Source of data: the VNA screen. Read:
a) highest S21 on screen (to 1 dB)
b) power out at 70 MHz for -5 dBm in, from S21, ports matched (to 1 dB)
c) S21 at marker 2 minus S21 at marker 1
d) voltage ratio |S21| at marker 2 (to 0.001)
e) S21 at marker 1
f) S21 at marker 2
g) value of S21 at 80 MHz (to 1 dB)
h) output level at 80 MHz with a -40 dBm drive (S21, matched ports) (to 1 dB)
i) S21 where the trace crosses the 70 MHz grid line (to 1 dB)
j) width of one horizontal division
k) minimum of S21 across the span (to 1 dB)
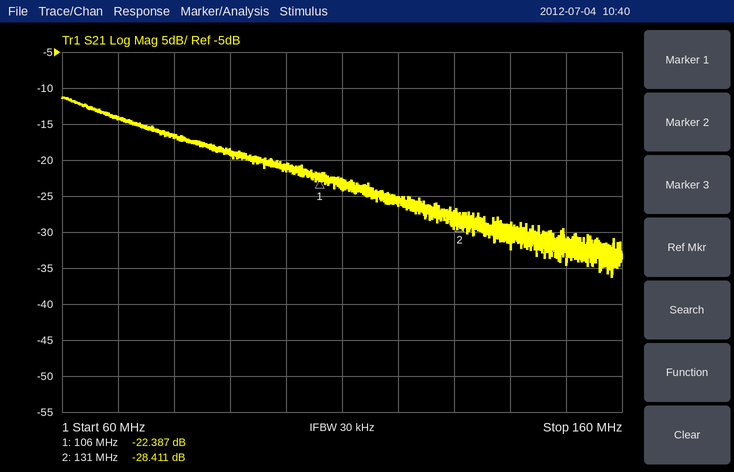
-11 dB
-19 dBm
-6.024 dB
0.038
-22.387 dB
-28.411 dB
-17 dB
-57 dBm
-14 dB
10 MHz
-36 dB
